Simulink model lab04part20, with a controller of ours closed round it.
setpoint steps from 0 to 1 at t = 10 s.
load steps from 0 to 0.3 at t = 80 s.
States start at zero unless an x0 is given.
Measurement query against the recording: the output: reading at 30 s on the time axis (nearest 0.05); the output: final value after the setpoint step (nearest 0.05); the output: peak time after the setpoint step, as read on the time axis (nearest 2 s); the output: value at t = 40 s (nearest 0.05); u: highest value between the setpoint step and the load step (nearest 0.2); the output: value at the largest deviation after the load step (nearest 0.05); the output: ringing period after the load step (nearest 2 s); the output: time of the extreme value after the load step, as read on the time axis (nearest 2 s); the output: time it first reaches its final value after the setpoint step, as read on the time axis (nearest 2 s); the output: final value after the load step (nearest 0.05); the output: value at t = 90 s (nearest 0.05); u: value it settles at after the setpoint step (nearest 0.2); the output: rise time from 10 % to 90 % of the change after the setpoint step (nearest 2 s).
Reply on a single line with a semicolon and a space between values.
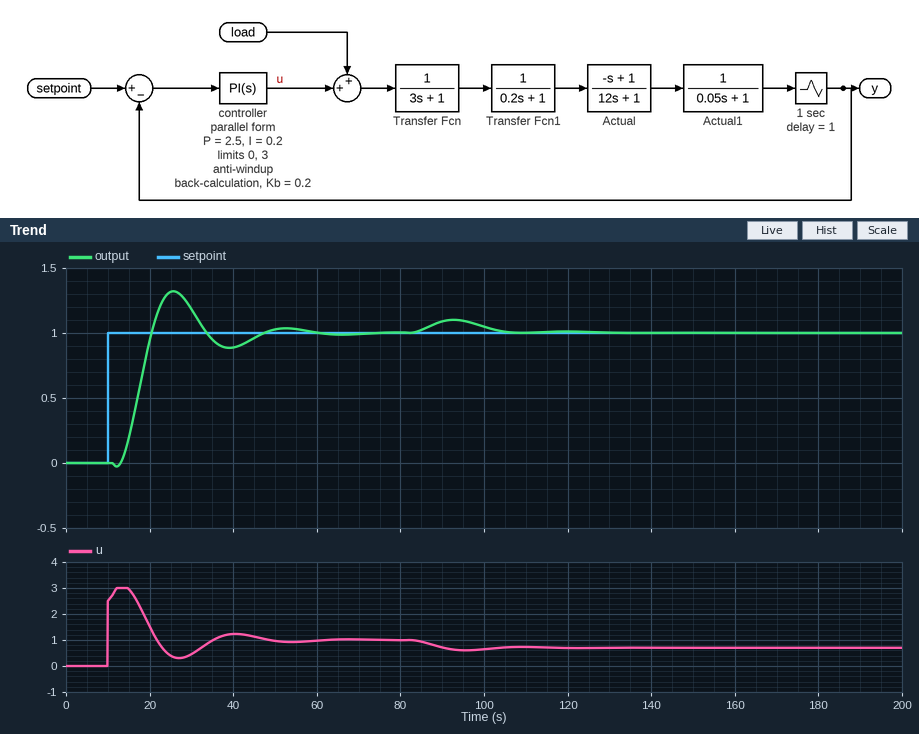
1.20; 1.00; 26 s; 0.90; 3.0; 1.10; 26 s; 92 s; 20 s; 1.00; 1.10; 1.0; 6 s
